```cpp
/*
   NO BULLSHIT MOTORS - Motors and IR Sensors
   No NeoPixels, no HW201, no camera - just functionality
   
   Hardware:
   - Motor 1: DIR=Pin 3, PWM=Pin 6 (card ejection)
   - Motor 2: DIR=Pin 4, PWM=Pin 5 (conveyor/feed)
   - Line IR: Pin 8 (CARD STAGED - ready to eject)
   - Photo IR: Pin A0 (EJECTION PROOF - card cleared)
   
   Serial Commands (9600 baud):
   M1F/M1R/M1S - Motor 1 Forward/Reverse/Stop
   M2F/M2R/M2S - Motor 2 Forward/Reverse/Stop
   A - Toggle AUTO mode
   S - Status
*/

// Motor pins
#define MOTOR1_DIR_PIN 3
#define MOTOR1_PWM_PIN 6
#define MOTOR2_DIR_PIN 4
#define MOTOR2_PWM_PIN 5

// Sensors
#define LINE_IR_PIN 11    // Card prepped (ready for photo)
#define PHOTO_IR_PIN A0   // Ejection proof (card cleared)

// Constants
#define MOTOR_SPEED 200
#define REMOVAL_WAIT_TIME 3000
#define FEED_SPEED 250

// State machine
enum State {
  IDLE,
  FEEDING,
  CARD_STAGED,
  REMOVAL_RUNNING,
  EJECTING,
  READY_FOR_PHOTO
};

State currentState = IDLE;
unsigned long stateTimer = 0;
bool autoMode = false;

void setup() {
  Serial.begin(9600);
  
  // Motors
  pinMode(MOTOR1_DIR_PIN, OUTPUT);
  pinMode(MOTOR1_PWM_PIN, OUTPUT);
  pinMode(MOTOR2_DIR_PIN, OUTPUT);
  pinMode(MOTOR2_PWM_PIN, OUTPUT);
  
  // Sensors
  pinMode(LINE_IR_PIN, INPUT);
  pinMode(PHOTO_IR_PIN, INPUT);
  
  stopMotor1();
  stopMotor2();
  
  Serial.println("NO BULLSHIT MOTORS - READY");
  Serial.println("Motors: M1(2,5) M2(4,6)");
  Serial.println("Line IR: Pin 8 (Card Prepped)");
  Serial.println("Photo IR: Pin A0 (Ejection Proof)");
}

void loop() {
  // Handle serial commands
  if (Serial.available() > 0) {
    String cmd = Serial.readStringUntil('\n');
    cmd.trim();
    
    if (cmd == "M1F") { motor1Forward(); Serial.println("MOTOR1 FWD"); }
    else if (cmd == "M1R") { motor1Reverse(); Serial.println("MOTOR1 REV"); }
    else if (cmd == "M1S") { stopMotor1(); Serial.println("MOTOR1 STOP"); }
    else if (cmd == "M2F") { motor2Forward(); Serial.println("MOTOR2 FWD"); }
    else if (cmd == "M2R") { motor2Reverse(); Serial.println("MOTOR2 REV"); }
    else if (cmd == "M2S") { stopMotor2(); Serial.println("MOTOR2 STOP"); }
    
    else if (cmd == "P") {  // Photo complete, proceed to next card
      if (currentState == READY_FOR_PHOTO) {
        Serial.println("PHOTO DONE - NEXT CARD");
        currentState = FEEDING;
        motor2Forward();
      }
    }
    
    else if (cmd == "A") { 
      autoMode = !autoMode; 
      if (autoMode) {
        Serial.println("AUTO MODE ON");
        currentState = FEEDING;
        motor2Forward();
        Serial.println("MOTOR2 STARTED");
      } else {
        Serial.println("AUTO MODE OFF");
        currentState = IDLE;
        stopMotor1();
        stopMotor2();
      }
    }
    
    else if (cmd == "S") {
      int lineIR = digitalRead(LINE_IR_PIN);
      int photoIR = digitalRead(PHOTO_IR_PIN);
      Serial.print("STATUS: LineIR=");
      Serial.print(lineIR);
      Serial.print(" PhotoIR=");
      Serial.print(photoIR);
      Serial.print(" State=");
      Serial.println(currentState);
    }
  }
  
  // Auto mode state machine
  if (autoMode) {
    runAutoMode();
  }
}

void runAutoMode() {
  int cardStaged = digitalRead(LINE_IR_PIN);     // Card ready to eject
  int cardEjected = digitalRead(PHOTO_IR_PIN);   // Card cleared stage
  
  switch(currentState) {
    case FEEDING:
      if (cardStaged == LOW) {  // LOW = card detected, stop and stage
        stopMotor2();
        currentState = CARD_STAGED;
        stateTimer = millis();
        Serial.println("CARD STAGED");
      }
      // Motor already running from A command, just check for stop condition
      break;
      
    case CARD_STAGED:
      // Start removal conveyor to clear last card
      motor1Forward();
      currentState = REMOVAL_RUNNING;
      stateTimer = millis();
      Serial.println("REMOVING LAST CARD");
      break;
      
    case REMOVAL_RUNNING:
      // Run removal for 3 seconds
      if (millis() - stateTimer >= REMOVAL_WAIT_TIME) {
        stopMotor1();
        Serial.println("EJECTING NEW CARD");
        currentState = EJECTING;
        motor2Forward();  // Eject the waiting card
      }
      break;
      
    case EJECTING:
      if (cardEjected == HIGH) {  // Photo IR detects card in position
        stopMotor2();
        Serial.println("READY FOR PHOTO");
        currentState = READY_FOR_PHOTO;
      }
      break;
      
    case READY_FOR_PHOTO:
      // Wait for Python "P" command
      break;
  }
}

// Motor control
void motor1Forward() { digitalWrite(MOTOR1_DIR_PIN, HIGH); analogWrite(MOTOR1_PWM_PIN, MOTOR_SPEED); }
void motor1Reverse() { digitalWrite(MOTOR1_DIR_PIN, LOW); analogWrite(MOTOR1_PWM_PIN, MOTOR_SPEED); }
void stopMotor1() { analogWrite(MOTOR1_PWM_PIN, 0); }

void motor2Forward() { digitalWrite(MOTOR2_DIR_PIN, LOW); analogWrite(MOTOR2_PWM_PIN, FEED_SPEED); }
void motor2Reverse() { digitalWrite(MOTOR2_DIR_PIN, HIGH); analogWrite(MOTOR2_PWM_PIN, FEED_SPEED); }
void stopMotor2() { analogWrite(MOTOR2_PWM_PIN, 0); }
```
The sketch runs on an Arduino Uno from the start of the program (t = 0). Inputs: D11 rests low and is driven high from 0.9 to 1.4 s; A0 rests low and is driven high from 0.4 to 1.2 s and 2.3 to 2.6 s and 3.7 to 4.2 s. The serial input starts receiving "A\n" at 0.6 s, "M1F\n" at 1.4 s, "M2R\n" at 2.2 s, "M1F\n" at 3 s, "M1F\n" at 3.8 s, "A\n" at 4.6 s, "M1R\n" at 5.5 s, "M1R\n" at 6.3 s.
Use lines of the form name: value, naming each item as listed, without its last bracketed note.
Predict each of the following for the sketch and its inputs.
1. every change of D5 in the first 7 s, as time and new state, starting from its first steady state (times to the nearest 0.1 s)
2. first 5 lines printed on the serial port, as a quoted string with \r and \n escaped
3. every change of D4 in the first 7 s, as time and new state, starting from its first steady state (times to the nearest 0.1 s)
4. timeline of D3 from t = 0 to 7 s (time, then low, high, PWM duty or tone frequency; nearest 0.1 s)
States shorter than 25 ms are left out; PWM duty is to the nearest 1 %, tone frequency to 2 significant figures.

every change of D5 in the first 7 s, as time and new state, starting from its first steady state: 0 s low; 2.2 s PWM 98 %; 3.7 s low
first 5 lines printed on the serial port, as a quoted string with \r and \n escaped: "NO BULLSHIT MOTORS - READY\r\nMotors: M1(2,5) M2(4,6)\r\nLine IR: Pin 8 (Card Prepped)\r\nPhoto IR: Pin A0 (Ejection Proof)\r\nAUTO MODE ON\r\n"
every change of D4 in the first 7 s, as time and new state, starting from its first steady state: 0 s low; 2.2 s high; 3.6 s low
timeline of D3 from t = 0 to 7 s: 0 s low; 0.6 s high; 5.5 s low
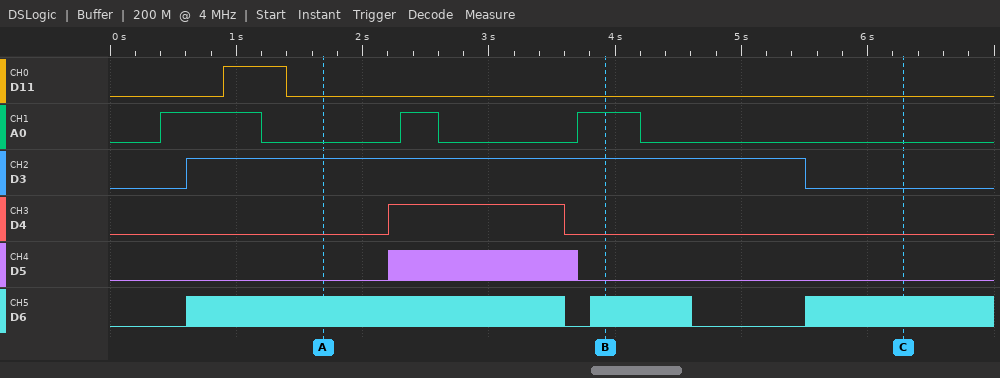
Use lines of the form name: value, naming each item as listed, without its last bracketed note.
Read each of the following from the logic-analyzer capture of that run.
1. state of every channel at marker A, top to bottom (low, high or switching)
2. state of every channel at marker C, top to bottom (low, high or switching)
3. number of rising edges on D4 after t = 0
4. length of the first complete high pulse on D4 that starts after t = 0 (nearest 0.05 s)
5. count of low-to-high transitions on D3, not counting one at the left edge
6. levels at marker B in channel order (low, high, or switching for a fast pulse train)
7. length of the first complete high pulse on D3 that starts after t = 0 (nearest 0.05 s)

state of every channel at marker A, top to bottom: D11 low, A0 low, D3 high, D4 low, D5 low, D6 switching
state of every channel at marker C, top to bottom: D11 low, A0 low, D3 low, D4 low, D5 low, D6 switching
number of rising edges on D4 after t = 0: 1
length of the first complete high pulse on D4 that starts after t = 0: 1.40 s
count of low-to-high transitions on D3, not counting one at the left edge: 1
levels at marker B in channel order: D11 low, A0 high, D3 high, D4 low, D5 low, D6 switching
length of the first complete high pulse on D3 that starts after t = 0: 4.90 s
